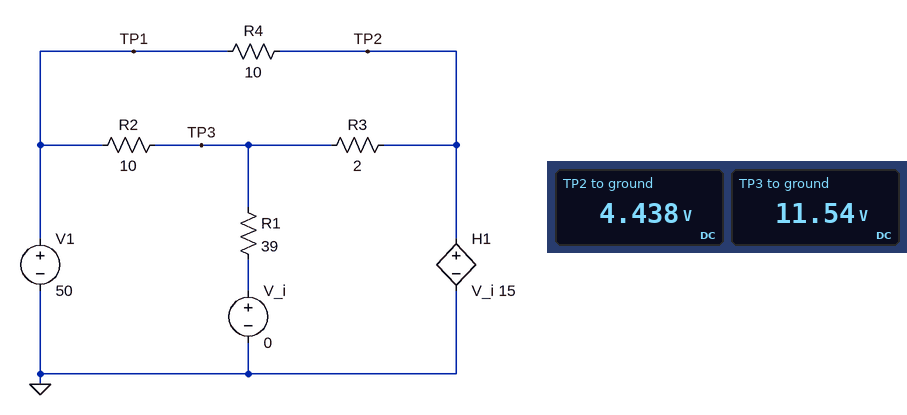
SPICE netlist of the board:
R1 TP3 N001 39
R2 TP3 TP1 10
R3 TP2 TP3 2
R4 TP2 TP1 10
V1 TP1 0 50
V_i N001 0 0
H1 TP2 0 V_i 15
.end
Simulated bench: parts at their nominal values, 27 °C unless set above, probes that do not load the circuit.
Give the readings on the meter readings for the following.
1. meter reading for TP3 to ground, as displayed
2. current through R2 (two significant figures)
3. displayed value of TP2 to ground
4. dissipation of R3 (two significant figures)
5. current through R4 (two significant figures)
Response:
11.54 V
3.8 A
4.438 V
25 W
4.6 A
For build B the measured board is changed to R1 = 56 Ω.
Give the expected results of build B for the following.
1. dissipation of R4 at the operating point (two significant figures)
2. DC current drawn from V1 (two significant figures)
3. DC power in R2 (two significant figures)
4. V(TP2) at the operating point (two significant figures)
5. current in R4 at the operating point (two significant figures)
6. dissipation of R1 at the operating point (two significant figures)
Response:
220 W
8.7 A
160 W
2.8 V
4.7 A
1.9 W
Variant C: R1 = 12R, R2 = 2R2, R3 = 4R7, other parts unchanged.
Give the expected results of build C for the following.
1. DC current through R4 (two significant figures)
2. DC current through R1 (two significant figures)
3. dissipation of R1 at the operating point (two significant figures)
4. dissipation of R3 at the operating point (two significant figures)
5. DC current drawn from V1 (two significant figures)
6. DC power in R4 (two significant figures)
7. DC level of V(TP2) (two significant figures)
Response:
860 mA
3.9 A
180 W
29 W
550 mA
7.4 W
59 V
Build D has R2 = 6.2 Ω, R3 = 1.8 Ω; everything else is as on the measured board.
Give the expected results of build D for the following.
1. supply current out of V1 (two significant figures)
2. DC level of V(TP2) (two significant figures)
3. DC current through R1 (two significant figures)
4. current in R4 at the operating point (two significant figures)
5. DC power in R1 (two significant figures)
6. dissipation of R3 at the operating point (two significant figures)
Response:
10 A
5.9 V
390 mA
4.4 A
6.0 W
49 W
